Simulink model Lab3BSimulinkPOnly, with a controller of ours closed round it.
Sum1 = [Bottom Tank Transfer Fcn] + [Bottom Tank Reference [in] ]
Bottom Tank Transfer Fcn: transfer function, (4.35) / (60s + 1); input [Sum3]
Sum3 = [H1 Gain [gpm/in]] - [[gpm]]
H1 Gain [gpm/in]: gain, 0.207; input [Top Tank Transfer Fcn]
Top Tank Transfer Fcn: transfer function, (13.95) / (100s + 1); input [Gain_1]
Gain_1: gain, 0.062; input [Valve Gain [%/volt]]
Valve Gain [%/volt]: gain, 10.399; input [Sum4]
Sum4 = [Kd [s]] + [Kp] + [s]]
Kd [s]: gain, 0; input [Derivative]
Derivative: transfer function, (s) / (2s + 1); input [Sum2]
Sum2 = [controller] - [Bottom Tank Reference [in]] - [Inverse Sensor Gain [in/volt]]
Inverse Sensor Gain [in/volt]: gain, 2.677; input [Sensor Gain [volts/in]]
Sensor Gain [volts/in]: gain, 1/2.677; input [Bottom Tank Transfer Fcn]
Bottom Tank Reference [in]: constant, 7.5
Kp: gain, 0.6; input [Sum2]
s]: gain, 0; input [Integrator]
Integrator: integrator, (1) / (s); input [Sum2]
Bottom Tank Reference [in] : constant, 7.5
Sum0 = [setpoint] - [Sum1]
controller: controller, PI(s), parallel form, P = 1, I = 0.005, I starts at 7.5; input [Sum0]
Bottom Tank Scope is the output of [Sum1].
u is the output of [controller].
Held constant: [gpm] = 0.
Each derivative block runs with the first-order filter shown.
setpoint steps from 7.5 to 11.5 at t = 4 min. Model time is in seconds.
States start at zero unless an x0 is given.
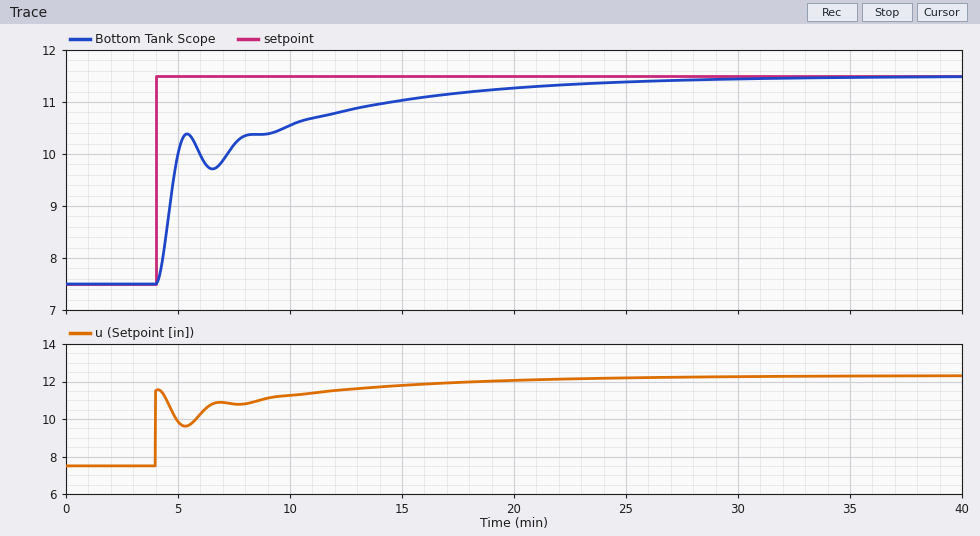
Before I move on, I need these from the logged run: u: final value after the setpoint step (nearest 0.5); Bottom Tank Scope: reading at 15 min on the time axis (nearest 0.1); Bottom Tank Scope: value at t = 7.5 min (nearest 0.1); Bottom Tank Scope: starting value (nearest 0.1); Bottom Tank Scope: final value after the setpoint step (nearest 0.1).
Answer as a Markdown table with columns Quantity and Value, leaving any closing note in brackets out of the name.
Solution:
| Quantity | Value |
|---|---|
| u: final value after the setpoint step | 12.5 |
| Bottom Tank Scope: reading at 15 min on the time axis | 11.0 |
| Bottom Tank Scope: value at t = 7.5 min | 10.2 |
| Bottom Tank Scope: starting value | 7.5 |
| Bottom Tank Scope: final value after the setpoint step | 11.5 |
